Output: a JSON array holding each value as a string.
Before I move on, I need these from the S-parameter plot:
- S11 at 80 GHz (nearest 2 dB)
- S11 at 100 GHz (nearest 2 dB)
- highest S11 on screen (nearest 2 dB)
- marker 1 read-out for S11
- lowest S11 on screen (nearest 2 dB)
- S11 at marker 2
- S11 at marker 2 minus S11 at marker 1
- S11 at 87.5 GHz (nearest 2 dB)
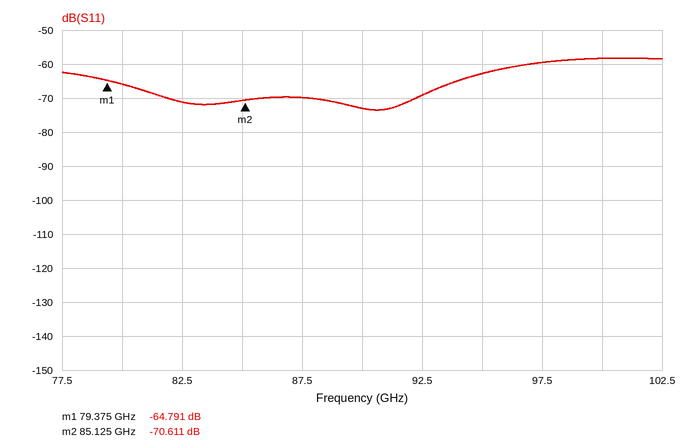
["-66 dB", "-58 dB", "-58 dB", "-64.791 dB", "-74 dB", "-70.611 dB", "-5.820 dB", "-70 dB"]
